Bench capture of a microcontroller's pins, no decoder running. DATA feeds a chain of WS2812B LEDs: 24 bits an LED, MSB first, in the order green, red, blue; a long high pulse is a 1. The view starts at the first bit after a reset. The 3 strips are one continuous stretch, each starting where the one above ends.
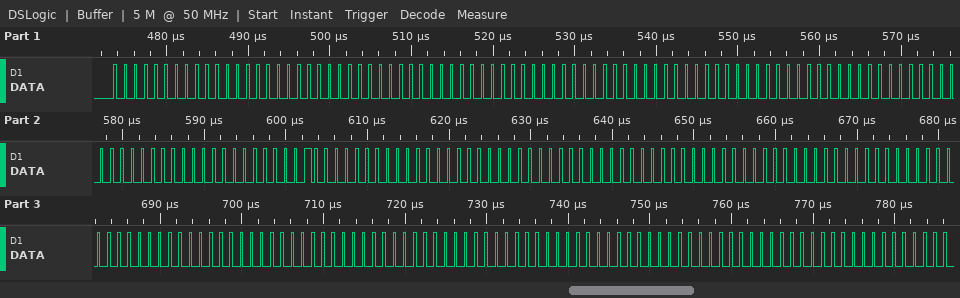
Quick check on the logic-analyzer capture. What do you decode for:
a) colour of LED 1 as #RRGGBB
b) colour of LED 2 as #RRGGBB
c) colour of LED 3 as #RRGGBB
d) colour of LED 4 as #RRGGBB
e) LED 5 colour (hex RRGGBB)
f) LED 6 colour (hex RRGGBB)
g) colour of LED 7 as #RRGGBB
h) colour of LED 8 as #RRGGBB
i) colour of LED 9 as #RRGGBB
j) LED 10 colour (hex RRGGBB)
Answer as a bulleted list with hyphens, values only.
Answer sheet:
- #000000
- #000000
- #000000
- #000000
- #000100
- #000000
- #000000
- #000000
- #000000
- #000000
